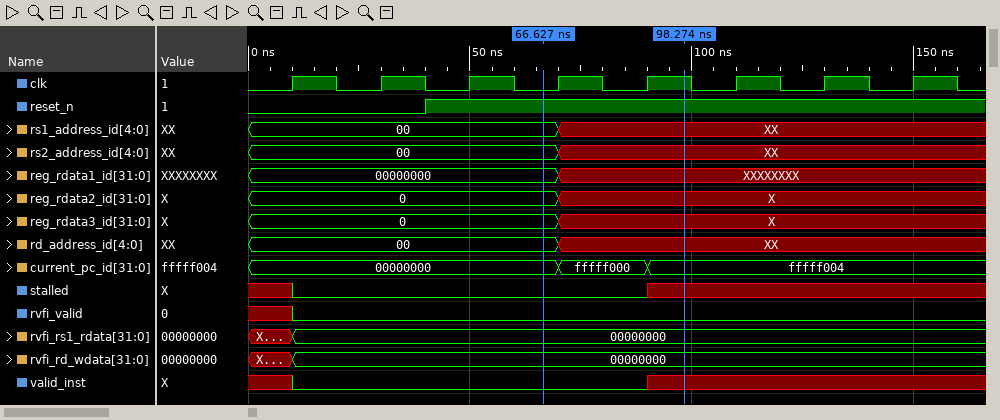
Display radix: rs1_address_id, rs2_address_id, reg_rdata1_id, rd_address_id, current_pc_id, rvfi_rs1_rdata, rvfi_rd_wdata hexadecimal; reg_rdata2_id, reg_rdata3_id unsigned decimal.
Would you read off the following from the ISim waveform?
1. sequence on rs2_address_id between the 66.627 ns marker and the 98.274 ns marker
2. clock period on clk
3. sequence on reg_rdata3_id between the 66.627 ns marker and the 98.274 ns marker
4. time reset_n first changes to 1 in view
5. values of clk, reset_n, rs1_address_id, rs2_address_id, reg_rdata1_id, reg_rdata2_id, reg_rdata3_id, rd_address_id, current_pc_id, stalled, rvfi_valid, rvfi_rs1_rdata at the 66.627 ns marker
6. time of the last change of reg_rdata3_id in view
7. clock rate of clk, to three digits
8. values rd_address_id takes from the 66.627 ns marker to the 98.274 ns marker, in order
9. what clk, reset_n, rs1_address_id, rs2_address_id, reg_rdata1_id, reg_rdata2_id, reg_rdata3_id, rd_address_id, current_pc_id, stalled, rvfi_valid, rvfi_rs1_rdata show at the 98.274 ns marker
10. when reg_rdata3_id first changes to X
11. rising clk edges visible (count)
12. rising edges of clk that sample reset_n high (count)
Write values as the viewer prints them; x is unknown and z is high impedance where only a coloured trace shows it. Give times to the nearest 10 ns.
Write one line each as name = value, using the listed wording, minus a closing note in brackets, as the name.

sequence on rs2_address_id between the 66.627 ns marker and the 98.274 ns marker = 00, XX
clock period on clk = 20 ns
sequence on reg_rdata3_id between the 66.627 ns marker and the 98.274 ns marker = 0, X
time reset_n first changes to 1 in view = 40 ns
values of clk, reset_n, rs1_address_id, rs2_address_id, reg_rdata1_id, reg_rdata2_id, reg_rdata3_id, rd_address_id, current_pc_id, stalled, rvfi_valid, rvfi_rs1_rdata at the 66.627 ns marker = clk=0, reset_n=1, rs1_address_id=00, rs2_address_id=00, reg_rdata1_id=00000000, reg_rdata2_id=0, reg_rdata3_id=0, rd_address_id=00, current_pc_id=00000000, stalled=0, rvfi_valid=0, rvfi_rs1_rdata=00000000
time of the last change of reg_rdata3_id in view = 70 ns
clock rate of clk, to three digits = 50.0 MHz
values rd_address_id takes from the 66.627 ns marker to the 98.274 ns marker, in order = 00, XX
what clk, reset_n, rs1_address_id, rs2_address_id, reg_rdata1_id, reg_rdata2_id, reg_rdata3_id, rd_address_id, current_pc_id, stalled, rvfi_valid, rvfi_rs1_rdata show at the 98.274 ns marker = clk=1, reset_n=1, rs1_address_id=XX, rs2_address_id=XX, reg_rdata1_id=XXXXXXXX, reg_rdata2_id=X, reg_rdata3_id=X, rd_address_id=XX, current_pc_id=fffff004, stalled=x, rvfi_valid=0, rvfi_rs1_rdata=00000000
when reg_rdata3_id first changes to X = 70 ns
rising clk edges visible = 8
rising edges of clk that sample reset_n high = 6
